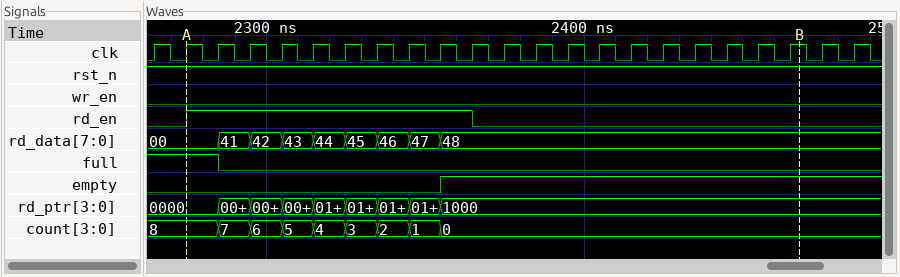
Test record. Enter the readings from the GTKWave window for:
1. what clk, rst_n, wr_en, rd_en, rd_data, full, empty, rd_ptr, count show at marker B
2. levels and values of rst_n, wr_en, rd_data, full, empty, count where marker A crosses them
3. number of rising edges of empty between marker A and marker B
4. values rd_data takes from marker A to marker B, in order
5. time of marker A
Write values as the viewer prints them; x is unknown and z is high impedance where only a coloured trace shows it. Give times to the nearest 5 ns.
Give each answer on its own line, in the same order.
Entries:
clk=1, rst_n=1, wr_en=0, rd_en=0, rd_data=48, full=0, empty=1, rd_ptr=1000, count=0
rst_n=1, wr_en=0, rd_data=00, full=1, empty=0, count=8
1
00, 41, 42, 43, 44, 45, 46, 47, 48
2275 ns
